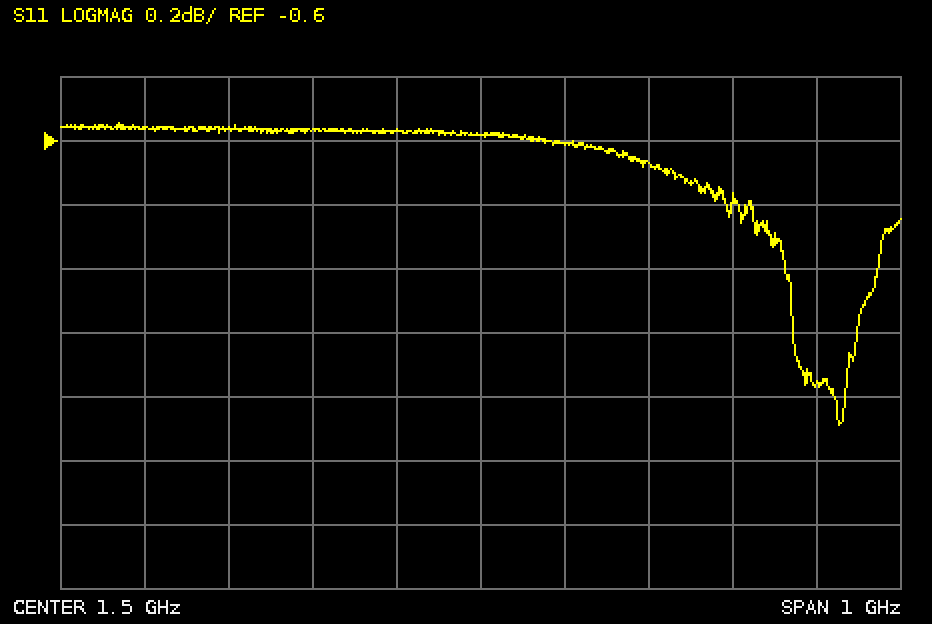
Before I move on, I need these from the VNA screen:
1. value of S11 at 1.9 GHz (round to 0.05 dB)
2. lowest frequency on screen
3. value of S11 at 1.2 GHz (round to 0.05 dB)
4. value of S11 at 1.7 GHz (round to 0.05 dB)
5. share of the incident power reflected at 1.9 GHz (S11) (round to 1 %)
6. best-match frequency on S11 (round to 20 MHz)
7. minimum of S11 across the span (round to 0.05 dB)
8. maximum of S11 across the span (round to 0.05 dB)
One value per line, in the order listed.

-1.35 dB
1 GHz
-0.55 dB
-0.65 dB
73 %
1.92 GHz
-1.50 dB
-0.55 dB
